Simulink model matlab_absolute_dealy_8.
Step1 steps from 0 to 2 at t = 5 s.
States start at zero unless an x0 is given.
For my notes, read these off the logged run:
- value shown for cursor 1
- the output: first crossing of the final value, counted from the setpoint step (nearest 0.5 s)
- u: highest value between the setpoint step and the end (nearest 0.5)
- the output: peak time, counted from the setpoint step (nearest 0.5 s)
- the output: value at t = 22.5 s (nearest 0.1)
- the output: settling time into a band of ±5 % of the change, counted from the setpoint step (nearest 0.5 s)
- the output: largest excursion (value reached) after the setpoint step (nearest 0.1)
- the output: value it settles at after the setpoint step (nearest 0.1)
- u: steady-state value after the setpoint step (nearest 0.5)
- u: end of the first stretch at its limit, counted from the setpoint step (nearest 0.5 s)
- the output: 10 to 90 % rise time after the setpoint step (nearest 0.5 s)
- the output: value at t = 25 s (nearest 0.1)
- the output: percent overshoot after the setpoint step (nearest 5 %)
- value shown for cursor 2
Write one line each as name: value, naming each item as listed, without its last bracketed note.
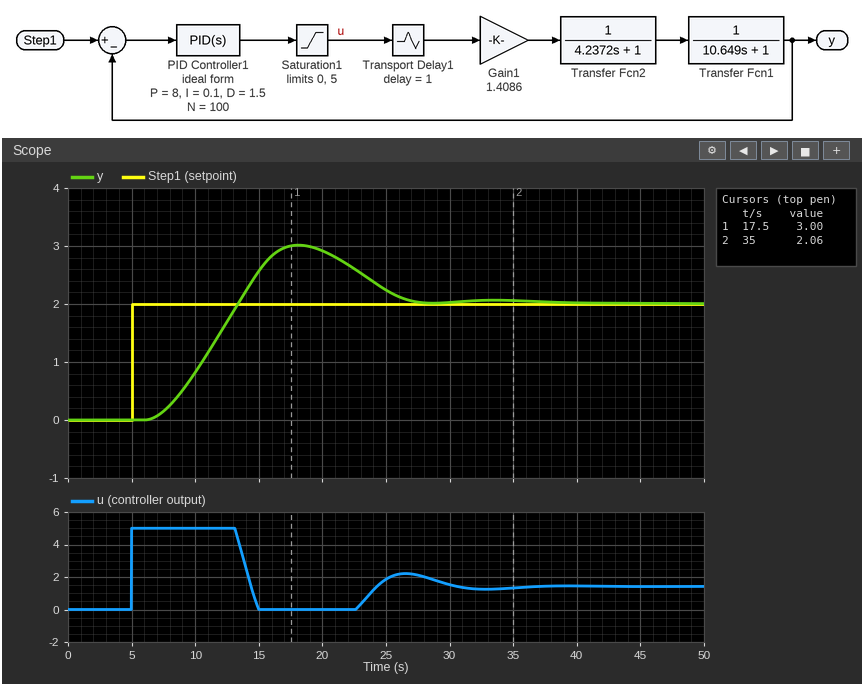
value shown for cursor 1: 3.00
the output: first crossing of the final value, counted from the setpoint step: 8.5 s
u: highest value between the setpoint step and the end: 5.0
the output: peak time, counted from the setpoint step: 13.0 s
the output: value at t = 22.5 s: 2.6
the output: settling time into a band of ±5 % of the change, counted from the setpoint step: 21.5 s
the output: largest excursion (value reached) after the setpoint step: 3.0
the output: value it settles at after the setpoint step: 2.0
u: steady-state value after the setpoint step: 1.5
u: end of the first stretch at its limit, counted from the setpoint step: 8.0 s
the output: 10 to 90 % rise time after the setpoint step: 5.0 s
the output: value at t = 25 s: 2.2
the output: percent overshoot after the setpoint step: 50 %
value shown for cursor 2: 2.06
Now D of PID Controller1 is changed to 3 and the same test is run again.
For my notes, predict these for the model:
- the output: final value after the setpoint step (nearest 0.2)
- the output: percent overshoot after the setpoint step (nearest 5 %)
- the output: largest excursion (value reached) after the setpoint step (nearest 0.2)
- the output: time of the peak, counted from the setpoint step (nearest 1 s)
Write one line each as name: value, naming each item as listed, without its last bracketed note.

the output: final value after the setpoint step: 2.0
the output: percent overshoot after the setpoint step: 35 %
the output: largest excursion (value reached) after the setpoint step: 2.6
the output: time of the peak, counted from the setpoint step: 14 s
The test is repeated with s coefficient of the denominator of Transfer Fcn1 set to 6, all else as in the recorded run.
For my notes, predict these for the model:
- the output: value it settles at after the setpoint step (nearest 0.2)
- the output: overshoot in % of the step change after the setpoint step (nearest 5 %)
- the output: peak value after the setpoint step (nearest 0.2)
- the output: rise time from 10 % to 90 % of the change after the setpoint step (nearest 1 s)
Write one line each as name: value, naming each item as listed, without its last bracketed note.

the output: value it settles at after the setpoint step: 2.0
the output: overshoot in % of the step change after the setpoint step: 40 %
the output: peak value after the setpoint step: 2.8
the output: rise time from 10 % to 90 % of the change after the setpoint step: 4 s
